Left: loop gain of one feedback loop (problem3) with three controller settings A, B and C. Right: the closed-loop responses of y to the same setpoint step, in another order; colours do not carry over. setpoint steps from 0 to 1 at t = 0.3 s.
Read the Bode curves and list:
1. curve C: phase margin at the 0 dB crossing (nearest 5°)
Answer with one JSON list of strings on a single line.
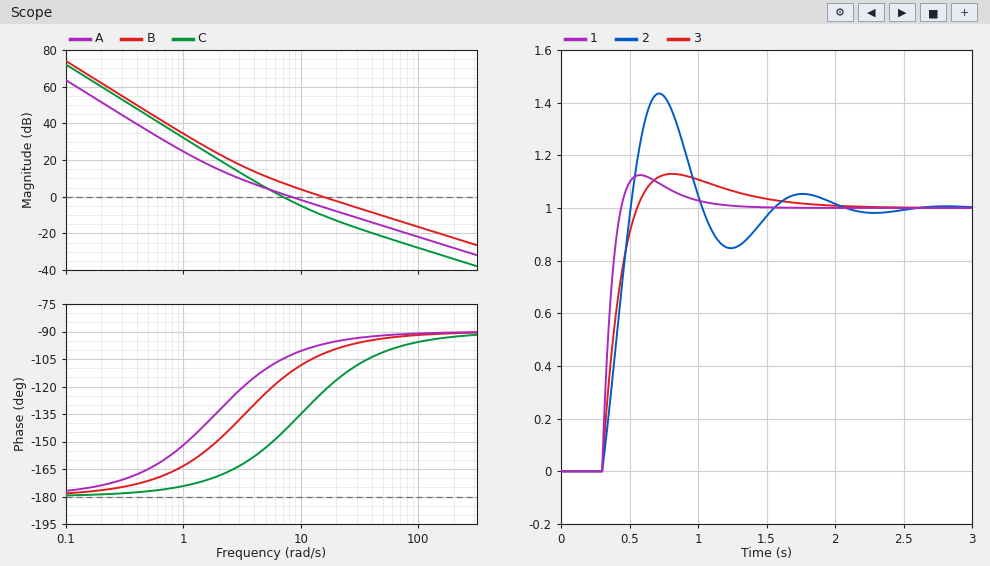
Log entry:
["35°"]
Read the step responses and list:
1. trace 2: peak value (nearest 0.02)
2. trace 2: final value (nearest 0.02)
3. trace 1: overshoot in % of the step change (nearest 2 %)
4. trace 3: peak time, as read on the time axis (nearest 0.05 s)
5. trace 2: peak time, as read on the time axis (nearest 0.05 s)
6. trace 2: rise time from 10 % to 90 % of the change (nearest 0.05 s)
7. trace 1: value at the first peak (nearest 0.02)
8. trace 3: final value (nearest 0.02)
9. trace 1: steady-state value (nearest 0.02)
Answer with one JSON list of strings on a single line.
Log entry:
["1.44", "1.00", "12 %", "0.80 s", "0.70 s", "0.15 s", "1.12", "1.00", "1.00"]
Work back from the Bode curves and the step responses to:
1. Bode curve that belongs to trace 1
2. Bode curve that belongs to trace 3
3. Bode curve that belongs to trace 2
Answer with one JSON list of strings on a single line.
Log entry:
["B", "A", "C"]
